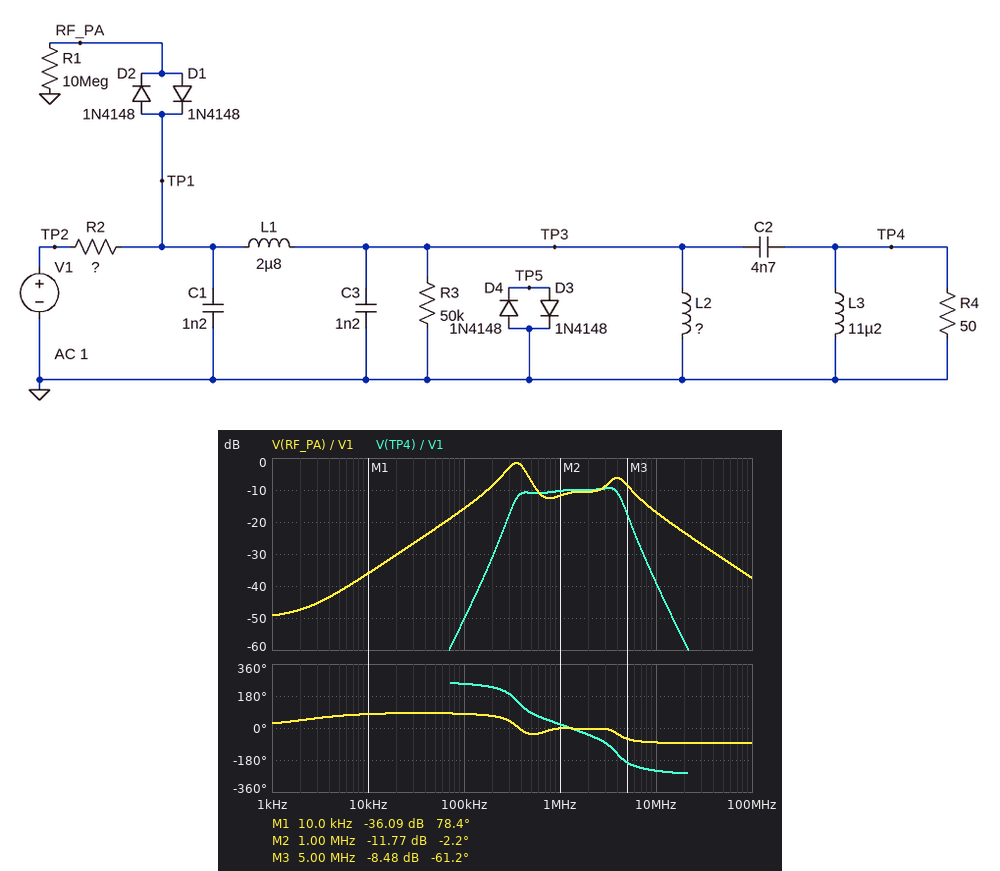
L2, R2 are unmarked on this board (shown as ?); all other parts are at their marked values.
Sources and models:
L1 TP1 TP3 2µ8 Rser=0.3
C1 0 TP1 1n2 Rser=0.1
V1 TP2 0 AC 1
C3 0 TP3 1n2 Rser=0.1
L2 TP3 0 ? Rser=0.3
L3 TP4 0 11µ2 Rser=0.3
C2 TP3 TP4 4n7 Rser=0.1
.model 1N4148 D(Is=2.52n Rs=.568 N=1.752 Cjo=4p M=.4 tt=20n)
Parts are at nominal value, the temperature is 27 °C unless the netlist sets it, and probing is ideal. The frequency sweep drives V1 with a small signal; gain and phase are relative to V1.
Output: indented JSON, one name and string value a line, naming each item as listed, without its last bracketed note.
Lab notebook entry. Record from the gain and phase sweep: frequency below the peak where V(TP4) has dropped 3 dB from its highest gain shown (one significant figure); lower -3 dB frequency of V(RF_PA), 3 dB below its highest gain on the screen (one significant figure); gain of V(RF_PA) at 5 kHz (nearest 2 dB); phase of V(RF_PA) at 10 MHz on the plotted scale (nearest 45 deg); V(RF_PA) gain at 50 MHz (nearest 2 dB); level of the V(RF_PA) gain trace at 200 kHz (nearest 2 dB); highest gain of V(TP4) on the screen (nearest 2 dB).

{
  "frequency below the peak where V(TP4) has dropped 3 dB from its highest gain shown": "400 kHz",
  "lower -3 dB frequency of V(RF_PA), 3 dB below its highest gain on the screen": "300 kHz",
  "gain of V(RF_PA) at 5 kHz": "-42 dB",
  "phase of V(RF_PA) at 10 MHz on the plotted scale": "-90 deg",
  "V(RF_PA) gain at 50 MHz": "-32 dB",
  "level of the V(RF_PA) gain trace at 200 kHz": "-8 dB",
  "highest gain of V(TP4) on the screen": "-10 dB"
}
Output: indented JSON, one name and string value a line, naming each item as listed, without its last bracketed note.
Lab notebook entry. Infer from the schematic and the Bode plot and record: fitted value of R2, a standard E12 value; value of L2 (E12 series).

{
  "fitted value of R2, a standard E12 value": "100 Ω",
  "value of L2": "22 µH"
}
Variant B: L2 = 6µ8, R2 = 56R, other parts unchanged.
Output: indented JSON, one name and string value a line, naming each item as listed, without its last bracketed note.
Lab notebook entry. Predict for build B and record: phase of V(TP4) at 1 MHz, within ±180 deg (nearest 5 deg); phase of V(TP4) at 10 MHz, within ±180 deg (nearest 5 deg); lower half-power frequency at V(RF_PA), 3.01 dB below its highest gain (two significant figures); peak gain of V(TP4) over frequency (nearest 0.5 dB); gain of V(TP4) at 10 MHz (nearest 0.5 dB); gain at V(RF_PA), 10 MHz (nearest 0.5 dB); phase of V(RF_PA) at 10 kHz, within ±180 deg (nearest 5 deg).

{
  "phase of V(TP4) at 1 MHz, within ±180 deg": "40 deg",
  "phase of V(TP4) at 10 MHz, within ±180 deg": "125 deg",
  "lower half-power frequency at V(RF_PA), 3.01 dB below its highest gain": "360 kHz",
  "peak gain of V(TP4) over frequency": "-6.5 dB",
  "gain of V(TP4) at 10 MHz": "-34.0 dB",
  "gain at V(RF_PA), 10 MHz": "-12.0 dB",
  "phase of V(RF_PA) at 10 kHz, within ±180 deg": "55 deg"
}
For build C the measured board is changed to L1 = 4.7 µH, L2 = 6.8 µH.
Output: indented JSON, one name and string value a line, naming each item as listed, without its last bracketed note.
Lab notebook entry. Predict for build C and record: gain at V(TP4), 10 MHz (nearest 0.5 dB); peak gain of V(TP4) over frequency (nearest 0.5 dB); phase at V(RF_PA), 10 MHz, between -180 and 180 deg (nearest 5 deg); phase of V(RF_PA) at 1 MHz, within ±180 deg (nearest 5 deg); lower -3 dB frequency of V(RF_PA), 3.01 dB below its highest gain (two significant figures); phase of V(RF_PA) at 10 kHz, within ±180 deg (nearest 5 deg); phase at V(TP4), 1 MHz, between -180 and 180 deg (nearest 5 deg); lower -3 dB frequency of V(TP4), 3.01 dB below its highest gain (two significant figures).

{
  "gain at V(TP4), 10 MHz": "-44.0 dB",
  "peak gain of V(TP4) over frequency": "-9.0 dB",
  "phase at V(RF_PA), 10 MHz, between -180 and 180 deg": "-80 deg",
  "phase of V(RF_PA) at 1 MHz, within ±180 deg": "15 deg",
  "lower -3 dB frequency of V(RF_PA), 3.01 dB below its highest gain": "400 kHz",
  "phase of V(RF_PA) at 10 kHz, within ±180 deg": "60 deg",
  "phase at V(TP4), 1 MHz, between -180 and 180 deg": "35 deg",
  "lower -3 dB frequency of V(TP4), 3.01 dB below its highest gain": "520 kHz"
}
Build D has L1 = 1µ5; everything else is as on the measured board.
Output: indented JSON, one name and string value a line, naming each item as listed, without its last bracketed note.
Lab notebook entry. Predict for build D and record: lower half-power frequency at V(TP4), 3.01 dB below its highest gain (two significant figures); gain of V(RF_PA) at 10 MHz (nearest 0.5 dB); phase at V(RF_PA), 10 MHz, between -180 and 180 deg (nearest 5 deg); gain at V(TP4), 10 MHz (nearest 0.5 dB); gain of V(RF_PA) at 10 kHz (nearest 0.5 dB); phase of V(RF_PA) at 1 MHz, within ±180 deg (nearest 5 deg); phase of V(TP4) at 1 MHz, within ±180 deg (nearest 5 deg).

{
  "lower half-power frequency at V(TP4), 3.01 dB below its highest gain": "350 kHz",
  "gain of V(RF_PA) at 10 MHz": "-16.0 dB",
  "phase at V(RF_PA), 10 MHz, between -180 and 180 deg": "-80 deg",
  "gain at V(TP4), 10 MHz": "-32.0 dB",
  "gain of V(RF_PA) at 10 kHz": "-36.5 dB",
  "phase of V(RF_PA) at 1 MHz, within ±180 deg": "-10 deg",
  "phase of V(TP4) at 1 MHz, within ±180 deg": "25 deg"
}
